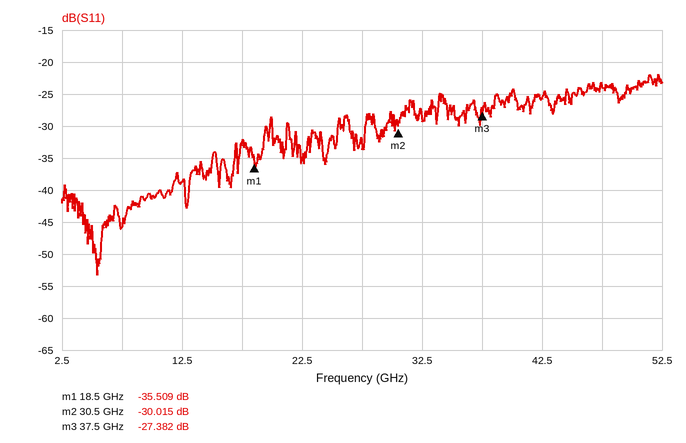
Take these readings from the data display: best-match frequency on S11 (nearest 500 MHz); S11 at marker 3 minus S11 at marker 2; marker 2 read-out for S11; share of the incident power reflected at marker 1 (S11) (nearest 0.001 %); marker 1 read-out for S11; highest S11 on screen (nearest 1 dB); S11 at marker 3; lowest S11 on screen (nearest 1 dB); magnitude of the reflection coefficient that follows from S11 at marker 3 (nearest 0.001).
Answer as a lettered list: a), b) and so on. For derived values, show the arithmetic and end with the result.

a) 5.5 GHz
b) -27.382 − (-30.015) = 2.633 dB
c) -30.015 dB
d) 10^(-35.509/10) ≈ 0.028 %
e) -35.509 dB
f) -22 dB
g) -27.382 dB
h) -53 dB
i) 10^(-27.382/20) ≈ 0.043
